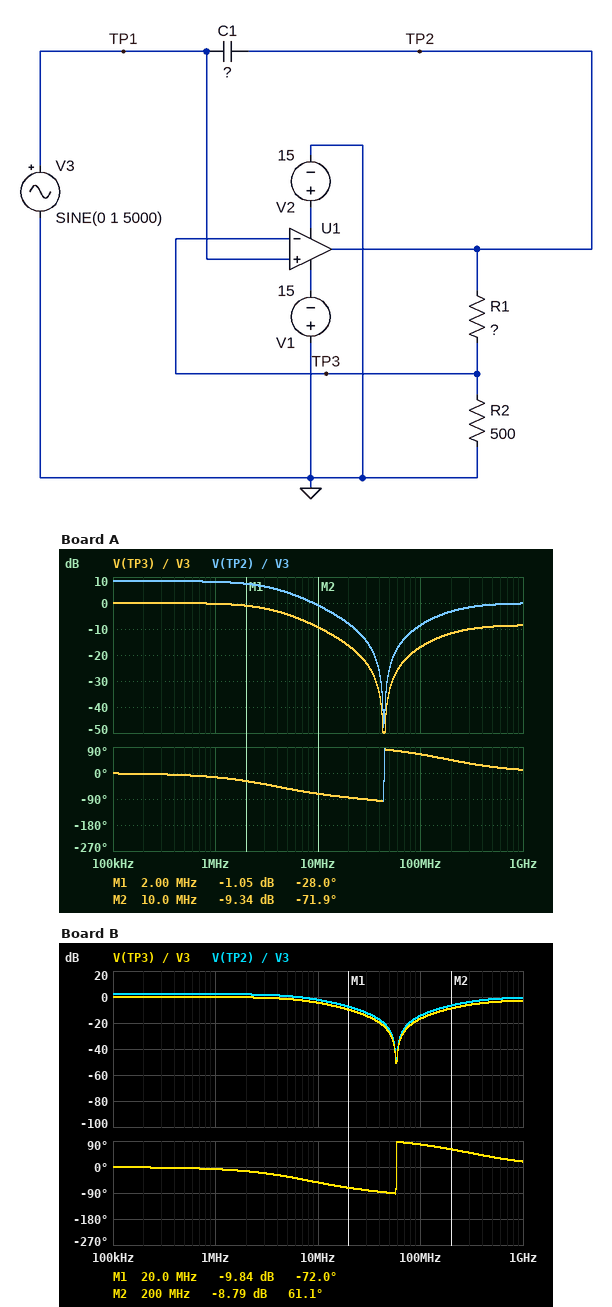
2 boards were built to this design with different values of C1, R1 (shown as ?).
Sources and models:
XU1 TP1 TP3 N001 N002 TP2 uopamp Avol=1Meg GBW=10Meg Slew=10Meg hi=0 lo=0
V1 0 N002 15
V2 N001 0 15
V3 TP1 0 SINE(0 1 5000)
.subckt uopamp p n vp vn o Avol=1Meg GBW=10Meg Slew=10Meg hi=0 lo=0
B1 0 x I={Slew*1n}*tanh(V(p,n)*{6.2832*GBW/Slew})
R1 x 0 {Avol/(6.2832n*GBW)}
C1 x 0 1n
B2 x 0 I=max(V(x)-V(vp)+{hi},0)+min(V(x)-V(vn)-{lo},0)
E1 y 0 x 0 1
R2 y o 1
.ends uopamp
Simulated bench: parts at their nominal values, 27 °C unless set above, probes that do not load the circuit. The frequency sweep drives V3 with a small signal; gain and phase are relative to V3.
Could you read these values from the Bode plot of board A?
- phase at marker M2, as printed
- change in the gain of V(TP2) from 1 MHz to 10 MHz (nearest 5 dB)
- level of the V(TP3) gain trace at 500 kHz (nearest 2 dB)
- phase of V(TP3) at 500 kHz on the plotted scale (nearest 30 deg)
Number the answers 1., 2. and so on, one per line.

1. -71.9 deg
2. -10 dB
3. 0 dB
4. 0 deg
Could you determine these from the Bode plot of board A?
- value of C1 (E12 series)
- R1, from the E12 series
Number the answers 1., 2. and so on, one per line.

1. 820 pF
2. 820 Ω
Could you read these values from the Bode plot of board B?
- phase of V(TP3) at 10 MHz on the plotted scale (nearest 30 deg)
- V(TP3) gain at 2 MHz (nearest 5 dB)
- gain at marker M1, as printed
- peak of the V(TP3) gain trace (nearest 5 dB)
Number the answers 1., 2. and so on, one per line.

1. -60 deg
2. 0 dB
3. -9.84 dB
4. 0 dB
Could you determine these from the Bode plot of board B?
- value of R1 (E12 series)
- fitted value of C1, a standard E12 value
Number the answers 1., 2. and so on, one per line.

1. 150 Ω
2. 470 pF
